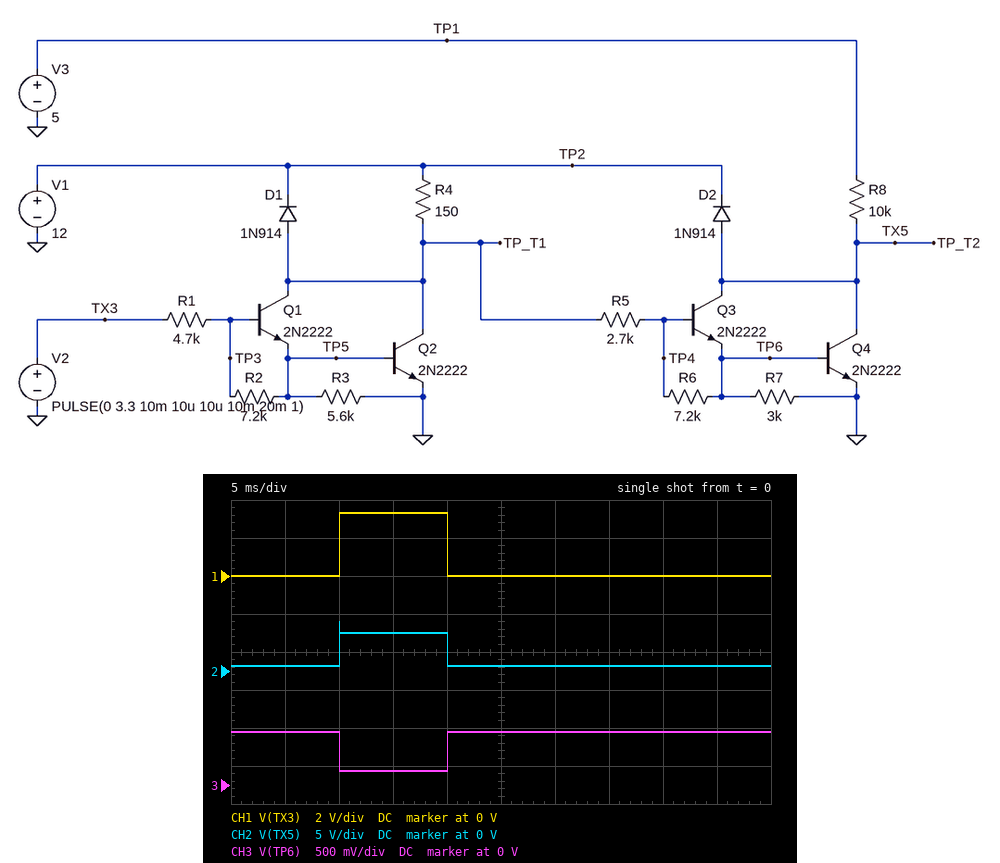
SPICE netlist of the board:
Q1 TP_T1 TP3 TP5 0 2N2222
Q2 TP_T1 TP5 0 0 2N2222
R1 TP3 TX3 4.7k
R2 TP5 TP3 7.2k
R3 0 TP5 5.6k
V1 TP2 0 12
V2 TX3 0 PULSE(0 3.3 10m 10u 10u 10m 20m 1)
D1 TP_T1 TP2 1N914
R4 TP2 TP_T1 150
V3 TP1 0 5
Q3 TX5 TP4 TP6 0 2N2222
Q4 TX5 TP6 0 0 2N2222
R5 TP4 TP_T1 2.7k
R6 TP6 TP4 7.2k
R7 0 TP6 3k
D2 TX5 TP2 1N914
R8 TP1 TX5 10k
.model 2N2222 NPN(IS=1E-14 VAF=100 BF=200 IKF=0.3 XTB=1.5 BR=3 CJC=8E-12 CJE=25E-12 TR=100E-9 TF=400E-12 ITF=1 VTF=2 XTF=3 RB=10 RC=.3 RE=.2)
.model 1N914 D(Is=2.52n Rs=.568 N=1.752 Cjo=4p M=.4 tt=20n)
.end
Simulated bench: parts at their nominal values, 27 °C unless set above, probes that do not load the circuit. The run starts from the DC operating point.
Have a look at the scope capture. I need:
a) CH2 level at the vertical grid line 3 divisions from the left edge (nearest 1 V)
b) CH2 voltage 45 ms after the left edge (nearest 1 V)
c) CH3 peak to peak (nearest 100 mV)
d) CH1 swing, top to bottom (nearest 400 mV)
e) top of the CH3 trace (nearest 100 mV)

5 V
1 V
500 mV
3.2 V
700 mV
